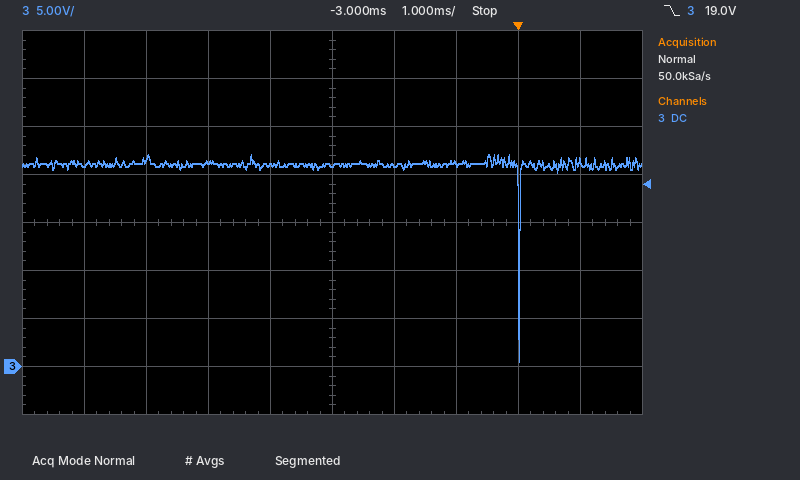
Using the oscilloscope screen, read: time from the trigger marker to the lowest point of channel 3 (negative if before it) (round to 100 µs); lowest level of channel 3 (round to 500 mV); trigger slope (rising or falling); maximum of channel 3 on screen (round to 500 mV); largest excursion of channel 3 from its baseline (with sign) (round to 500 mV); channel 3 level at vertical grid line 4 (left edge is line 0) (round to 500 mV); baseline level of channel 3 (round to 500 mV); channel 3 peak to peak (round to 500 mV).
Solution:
0.0 ms
500 mV
falling
22.0 V
-20.5 V
21.0 V
21.0 V
21.5 V
